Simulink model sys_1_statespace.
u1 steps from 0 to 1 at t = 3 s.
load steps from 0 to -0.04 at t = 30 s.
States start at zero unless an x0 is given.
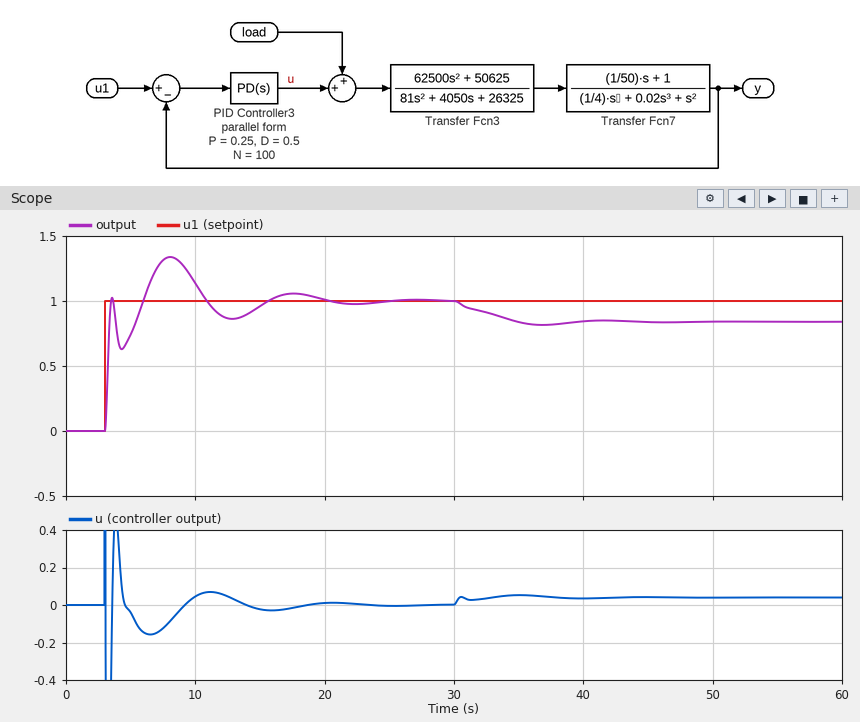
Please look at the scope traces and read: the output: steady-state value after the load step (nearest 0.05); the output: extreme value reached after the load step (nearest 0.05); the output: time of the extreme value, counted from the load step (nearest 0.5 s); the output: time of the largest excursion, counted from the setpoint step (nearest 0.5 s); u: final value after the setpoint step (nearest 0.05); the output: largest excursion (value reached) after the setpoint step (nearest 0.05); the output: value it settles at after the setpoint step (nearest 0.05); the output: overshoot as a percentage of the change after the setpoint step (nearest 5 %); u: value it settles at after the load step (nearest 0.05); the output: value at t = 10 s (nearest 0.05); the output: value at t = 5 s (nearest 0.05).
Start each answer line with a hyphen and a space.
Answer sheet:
- 0.85
- 0.80
- 7.0 s
- 5.0 s
- 0.00
- 1.35
- 1.00
- 35 %
- 0.05
- 1.15
- 0.75
